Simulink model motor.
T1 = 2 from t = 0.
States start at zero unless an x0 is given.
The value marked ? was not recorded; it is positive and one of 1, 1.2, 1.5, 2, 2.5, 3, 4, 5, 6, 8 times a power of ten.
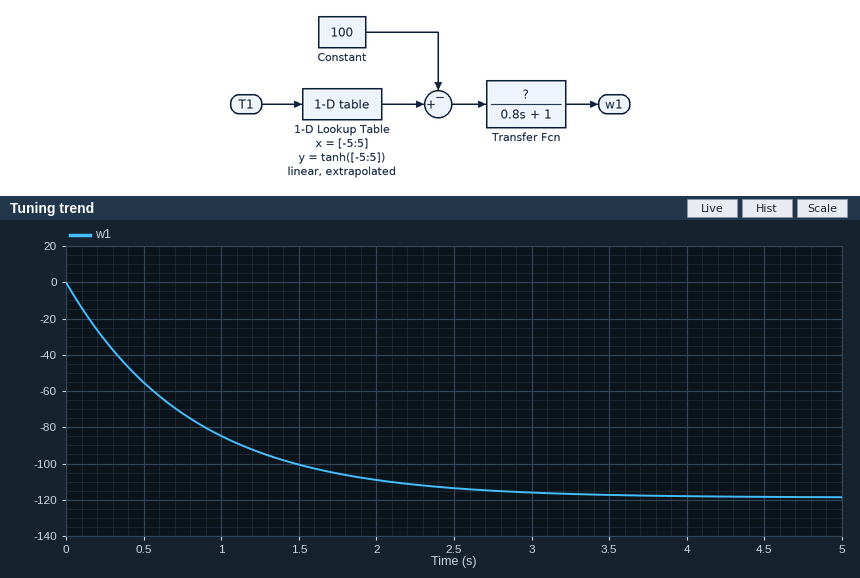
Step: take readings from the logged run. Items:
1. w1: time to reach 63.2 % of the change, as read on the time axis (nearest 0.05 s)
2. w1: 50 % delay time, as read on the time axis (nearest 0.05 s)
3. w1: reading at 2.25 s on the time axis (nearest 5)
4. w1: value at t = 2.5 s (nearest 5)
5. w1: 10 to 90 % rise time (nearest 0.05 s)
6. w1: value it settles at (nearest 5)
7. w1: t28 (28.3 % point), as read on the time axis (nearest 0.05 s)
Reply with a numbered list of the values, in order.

1. 0.80 s
2. 0.55 s
3. -110
4. -115
5. 1.75 s
6. -120
7. 0.25 s
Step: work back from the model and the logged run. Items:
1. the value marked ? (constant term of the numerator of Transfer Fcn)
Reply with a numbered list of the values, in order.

1. 1.2
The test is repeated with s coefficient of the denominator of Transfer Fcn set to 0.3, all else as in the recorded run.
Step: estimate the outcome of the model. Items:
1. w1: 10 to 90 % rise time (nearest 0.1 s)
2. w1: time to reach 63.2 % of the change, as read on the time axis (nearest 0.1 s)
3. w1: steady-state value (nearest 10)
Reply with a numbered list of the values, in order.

1. 0.7 s
2. 0.3 s
3. -120
